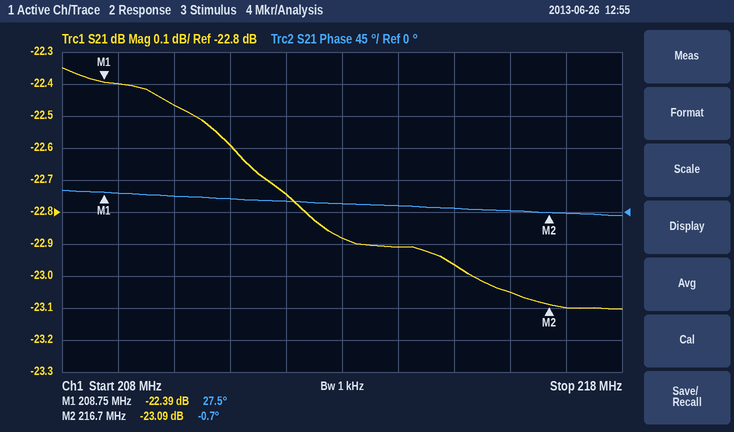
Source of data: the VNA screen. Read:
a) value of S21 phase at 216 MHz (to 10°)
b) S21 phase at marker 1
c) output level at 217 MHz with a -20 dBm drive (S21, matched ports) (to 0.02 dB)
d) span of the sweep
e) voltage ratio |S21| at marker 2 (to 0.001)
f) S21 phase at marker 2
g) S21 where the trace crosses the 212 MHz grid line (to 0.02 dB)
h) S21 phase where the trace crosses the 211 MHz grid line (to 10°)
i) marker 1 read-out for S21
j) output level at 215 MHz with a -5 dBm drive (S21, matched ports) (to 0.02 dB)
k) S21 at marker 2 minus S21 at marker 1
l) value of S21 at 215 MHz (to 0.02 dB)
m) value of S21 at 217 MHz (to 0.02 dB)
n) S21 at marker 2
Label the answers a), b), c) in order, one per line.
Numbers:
a) 0°
b) 27.5°
c) -43.10 dBm
d) 10 MHz
e) 0.070
f) -0.7°
g) -22.74 dB
h) 20°
i) -22.39 dB
j) -27.96 dBm
k) -0.70 dB
l) -22.96 dB
m) -23.10 dB
n) -23.09 dB
